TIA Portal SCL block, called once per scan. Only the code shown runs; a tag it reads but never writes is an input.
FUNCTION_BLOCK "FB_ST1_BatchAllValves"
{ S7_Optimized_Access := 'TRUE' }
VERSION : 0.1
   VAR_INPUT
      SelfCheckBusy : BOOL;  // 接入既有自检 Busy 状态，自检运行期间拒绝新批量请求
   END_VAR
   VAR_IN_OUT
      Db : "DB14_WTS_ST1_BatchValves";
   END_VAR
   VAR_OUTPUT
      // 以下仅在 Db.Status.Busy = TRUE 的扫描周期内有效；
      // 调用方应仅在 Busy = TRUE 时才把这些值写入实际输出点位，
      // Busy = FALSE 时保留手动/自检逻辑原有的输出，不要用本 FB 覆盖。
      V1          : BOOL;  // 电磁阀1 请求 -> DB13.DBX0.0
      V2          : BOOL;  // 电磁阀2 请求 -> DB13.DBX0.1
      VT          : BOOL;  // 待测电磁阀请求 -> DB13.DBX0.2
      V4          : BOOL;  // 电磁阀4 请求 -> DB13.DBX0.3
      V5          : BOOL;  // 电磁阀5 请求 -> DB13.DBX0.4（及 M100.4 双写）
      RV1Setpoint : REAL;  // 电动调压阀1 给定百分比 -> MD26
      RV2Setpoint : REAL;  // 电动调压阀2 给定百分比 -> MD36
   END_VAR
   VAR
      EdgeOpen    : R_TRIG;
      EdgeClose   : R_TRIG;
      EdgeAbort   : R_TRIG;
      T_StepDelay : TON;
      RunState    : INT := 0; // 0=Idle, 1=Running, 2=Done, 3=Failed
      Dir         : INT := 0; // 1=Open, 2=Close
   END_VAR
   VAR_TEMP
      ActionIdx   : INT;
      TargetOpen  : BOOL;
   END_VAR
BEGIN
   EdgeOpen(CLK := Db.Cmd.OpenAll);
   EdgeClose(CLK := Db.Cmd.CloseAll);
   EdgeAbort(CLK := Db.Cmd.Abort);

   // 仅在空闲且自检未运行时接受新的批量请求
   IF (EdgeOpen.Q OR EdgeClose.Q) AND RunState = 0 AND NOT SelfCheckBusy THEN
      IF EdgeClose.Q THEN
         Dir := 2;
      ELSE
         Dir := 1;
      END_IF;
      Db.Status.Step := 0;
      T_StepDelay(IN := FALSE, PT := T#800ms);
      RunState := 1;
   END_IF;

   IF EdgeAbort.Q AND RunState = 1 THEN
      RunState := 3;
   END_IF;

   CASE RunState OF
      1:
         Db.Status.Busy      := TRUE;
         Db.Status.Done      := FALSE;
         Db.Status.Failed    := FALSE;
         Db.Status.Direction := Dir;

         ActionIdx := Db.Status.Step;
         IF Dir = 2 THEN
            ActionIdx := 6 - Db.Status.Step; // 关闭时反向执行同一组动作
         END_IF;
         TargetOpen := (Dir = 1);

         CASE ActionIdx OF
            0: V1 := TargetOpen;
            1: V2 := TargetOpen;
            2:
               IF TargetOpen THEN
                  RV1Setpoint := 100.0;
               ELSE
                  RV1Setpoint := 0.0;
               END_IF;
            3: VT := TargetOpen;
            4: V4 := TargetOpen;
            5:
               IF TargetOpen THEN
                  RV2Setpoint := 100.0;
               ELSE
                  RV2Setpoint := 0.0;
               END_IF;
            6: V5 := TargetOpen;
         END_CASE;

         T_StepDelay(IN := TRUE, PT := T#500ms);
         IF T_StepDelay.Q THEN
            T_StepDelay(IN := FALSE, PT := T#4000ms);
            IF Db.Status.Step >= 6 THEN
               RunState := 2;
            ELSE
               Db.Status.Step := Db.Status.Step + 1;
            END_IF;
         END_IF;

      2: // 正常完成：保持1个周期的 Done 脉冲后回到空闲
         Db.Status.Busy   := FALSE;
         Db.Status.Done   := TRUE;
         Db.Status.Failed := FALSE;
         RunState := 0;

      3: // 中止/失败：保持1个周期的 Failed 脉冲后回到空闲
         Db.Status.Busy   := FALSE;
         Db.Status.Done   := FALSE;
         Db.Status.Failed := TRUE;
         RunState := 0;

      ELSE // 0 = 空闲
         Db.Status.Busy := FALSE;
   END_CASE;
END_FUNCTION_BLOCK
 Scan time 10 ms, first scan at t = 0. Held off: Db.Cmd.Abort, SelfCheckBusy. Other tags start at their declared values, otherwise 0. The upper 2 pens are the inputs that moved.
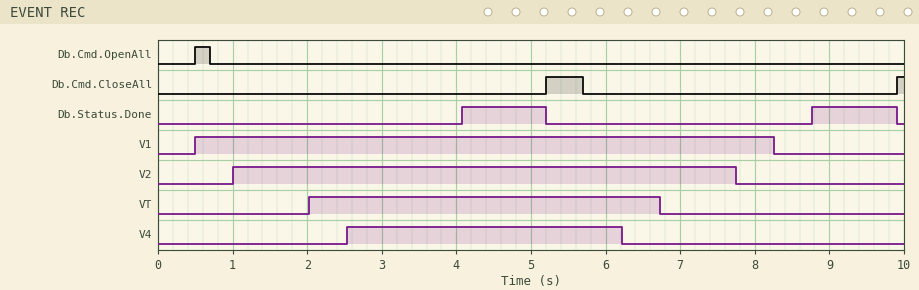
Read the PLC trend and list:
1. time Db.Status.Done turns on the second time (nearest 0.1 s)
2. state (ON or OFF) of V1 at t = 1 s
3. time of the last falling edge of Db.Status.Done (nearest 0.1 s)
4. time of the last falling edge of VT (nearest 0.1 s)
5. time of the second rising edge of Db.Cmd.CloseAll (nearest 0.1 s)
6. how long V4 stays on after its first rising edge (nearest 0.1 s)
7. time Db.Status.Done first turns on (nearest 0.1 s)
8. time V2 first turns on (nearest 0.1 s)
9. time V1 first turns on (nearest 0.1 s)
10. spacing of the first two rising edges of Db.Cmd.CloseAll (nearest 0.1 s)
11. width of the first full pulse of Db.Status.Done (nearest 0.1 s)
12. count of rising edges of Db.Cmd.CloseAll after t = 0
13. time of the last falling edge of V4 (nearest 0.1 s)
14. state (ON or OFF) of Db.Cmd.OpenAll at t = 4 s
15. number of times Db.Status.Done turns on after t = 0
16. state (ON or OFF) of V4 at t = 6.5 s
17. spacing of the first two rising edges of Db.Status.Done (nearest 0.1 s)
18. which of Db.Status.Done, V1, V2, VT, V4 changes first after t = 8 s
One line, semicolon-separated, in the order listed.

8.8 s; ON; 9.9 s; 6.7 s; 9.9 s; 3.7 s; 4.1 s; 1.0 s; 0.5 s; 4.7 s; 1.1 s; 2; 6.2 s; OFF; 2; OFF; 4.7 s; V1
